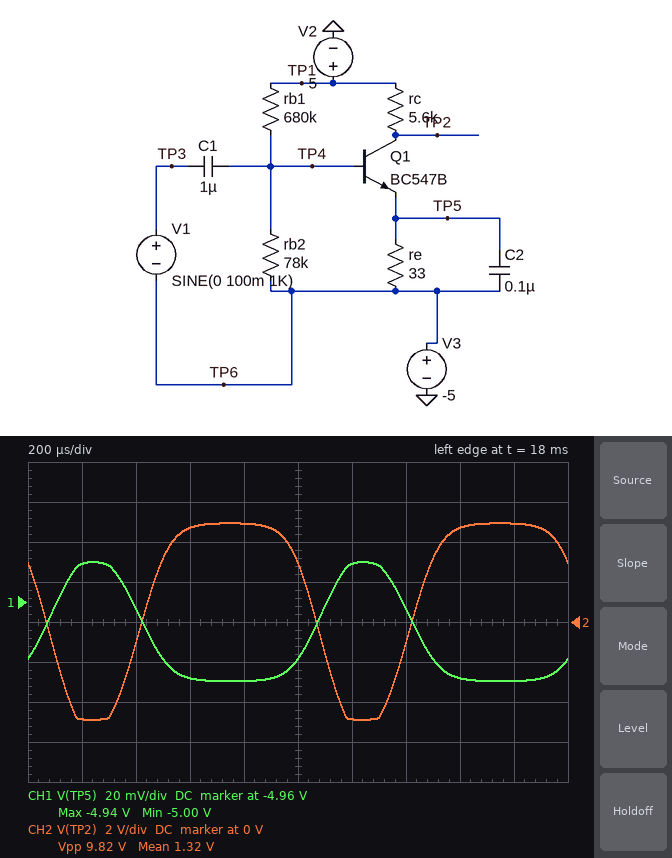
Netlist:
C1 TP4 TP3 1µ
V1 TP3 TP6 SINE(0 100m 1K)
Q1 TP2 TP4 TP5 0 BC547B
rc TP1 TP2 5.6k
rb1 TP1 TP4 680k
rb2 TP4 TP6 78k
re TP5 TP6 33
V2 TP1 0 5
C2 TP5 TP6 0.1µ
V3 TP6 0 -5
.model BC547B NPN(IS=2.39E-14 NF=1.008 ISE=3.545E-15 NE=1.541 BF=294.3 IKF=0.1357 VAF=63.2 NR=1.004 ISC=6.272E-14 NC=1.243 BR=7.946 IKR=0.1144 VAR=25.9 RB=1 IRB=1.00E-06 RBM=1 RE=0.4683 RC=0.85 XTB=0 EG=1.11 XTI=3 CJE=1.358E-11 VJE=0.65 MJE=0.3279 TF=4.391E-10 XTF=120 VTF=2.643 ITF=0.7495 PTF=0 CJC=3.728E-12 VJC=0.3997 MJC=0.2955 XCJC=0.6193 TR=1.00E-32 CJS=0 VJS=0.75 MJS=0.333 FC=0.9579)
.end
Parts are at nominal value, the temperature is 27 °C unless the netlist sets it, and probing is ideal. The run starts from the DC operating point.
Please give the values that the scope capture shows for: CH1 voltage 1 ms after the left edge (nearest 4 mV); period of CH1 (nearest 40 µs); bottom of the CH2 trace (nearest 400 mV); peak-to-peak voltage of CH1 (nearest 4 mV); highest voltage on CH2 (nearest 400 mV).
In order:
-4.988 V
1.00 ms
-4.8 V
60 mV
4.8 V
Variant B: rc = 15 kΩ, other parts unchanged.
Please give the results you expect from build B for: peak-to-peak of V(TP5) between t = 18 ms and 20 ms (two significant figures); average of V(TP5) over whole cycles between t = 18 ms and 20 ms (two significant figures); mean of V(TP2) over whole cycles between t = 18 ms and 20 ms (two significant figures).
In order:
24 mV
-5.0 V
1.7 V
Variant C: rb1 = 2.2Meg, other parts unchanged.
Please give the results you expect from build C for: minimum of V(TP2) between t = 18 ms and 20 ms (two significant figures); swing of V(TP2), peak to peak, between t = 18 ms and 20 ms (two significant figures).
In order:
5.0 V
3.5 mV
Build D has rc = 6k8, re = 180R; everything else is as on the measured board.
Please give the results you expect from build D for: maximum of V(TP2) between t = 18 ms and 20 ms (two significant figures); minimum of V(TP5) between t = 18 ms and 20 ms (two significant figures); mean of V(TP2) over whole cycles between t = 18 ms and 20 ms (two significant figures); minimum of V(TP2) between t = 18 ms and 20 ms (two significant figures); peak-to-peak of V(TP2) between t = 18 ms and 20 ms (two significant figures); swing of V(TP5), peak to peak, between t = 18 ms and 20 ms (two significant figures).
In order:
1.8 V
-4.9 V
-1.4 V
-4.6 V
6.4 V
170 mV
